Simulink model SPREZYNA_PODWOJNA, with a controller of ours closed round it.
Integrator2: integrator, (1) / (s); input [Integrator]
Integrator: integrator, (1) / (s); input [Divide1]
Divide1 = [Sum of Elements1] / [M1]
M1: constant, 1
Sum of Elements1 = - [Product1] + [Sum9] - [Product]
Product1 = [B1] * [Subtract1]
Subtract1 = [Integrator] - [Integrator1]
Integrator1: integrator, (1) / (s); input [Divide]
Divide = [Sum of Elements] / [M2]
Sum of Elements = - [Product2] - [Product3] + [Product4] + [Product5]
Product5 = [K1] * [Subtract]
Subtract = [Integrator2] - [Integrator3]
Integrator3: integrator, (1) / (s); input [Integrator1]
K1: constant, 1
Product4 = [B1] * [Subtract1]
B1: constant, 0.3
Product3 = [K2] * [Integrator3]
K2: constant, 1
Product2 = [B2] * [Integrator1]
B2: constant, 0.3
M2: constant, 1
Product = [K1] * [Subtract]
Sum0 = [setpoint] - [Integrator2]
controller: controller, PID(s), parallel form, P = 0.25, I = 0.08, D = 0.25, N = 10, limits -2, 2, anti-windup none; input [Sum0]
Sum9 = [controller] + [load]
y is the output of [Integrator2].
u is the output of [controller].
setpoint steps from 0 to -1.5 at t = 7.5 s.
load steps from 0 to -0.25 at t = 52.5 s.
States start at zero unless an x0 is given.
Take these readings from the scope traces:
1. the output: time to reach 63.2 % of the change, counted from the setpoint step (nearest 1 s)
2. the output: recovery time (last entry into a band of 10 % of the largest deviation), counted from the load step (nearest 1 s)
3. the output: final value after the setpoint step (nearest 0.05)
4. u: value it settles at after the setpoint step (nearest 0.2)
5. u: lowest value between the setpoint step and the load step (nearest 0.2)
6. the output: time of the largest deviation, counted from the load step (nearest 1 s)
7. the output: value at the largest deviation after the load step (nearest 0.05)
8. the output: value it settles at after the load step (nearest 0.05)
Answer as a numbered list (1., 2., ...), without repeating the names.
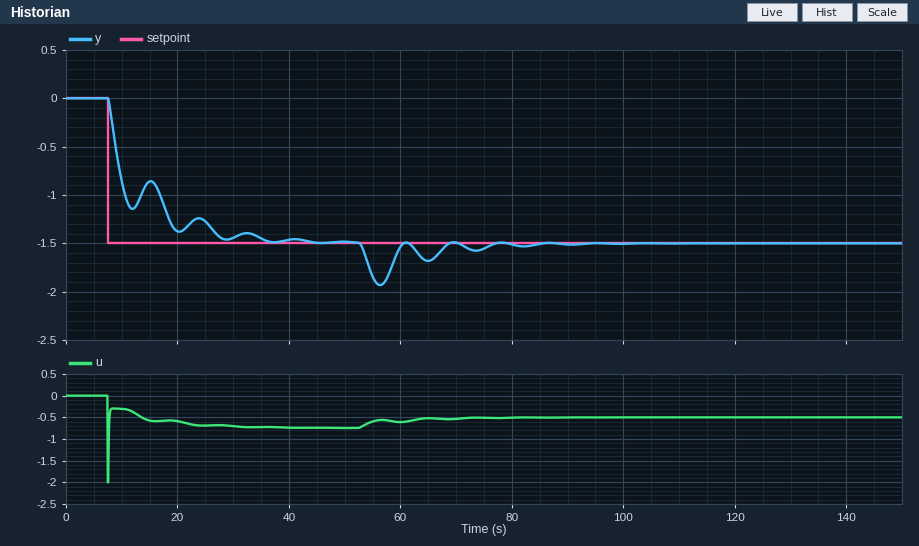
1. 3 s
2. 23 s
3. -1.50
4. -0.8
5. -2.0
6. 4 s
7. -1.95
8. -1.50
